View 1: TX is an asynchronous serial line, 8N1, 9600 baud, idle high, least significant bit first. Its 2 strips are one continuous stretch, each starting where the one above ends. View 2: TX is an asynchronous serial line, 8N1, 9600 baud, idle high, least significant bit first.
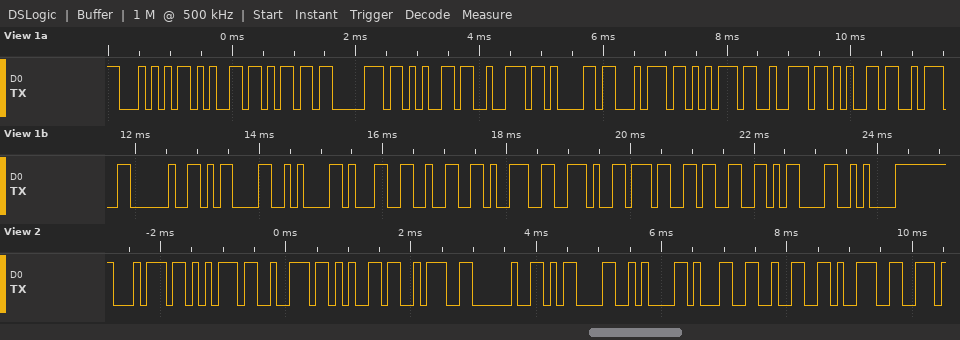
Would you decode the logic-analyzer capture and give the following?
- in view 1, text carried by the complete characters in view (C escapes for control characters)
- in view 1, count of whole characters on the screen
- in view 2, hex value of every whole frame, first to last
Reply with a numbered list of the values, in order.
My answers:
1. "Temperature: \r\n129.73\r\n"
2. 23
3. 0x74 0x75 0x72 0x65 0x3A 0x20 0x0D 0x0A 0x31 0x32 0x39
